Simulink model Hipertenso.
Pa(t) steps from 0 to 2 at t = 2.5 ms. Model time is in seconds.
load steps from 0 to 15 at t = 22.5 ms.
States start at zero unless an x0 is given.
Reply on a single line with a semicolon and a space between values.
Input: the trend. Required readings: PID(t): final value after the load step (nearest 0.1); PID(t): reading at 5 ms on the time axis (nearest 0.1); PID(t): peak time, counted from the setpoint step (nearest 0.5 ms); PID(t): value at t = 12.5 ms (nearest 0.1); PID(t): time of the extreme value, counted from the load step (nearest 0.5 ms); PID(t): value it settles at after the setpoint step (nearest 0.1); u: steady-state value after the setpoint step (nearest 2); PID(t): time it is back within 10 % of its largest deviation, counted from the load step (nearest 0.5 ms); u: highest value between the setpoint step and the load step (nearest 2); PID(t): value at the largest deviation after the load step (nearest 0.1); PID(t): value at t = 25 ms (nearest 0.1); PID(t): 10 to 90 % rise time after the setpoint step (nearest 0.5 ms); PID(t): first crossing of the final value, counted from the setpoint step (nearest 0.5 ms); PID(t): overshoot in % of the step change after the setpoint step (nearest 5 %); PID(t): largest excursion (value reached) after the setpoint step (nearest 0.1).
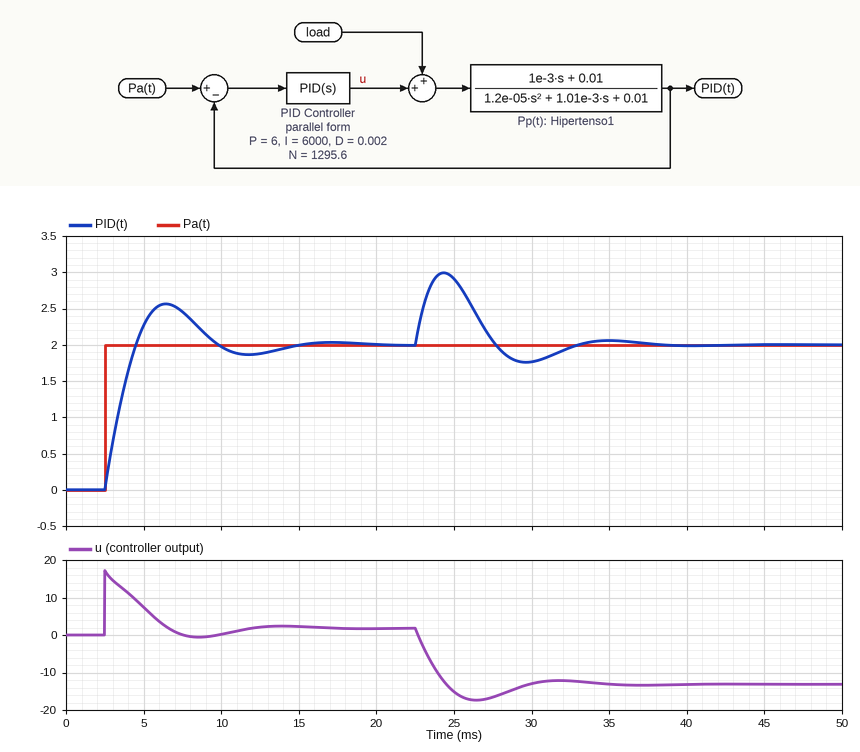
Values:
2.0; 2.3; 4.0 ms; 1.9; 2.0 ms; 2.0; 2; 9.5 ms; 18; 3.0; 2.9; 1.5 ms; 2.0 ms; 30 %; 2.6
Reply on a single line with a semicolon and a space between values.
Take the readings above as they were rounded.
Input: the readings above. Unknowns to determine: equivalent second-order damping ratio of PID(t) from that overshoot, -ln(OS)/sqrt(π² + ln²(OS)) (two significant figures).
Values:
0.36
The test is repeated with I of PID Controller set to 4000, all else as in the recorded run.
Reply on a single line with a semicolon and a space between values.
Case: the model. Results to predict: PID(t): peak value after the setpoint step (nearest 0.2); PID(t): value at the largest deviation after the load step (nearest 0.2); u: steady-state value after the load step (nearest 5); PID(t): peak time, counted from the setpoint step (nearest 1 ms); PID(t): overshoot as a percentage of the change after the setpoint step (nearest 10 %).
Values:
2.4; 3.2; -15; 5 ms; 20 %
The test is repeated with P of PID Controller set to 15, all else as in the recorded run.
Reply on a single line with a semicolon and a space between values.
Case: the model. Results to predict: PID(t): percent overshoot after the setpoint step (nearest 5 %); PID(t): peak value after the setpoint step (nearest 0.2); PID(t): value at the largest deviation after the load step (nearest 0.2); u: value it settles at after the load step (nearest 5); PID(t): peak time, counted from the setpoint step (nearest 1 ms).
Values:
10 %; 2.2; 2.6; -15; 3 ms
